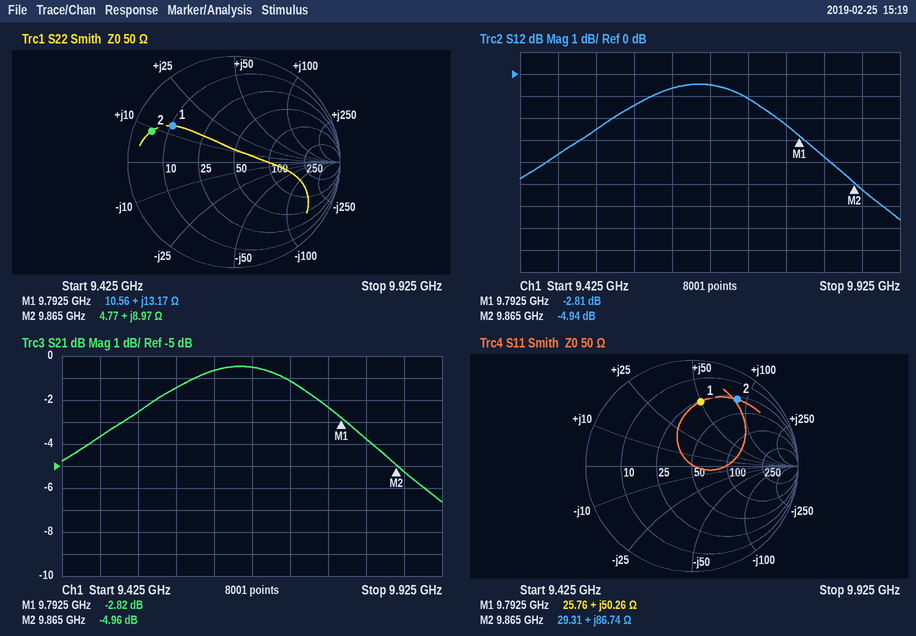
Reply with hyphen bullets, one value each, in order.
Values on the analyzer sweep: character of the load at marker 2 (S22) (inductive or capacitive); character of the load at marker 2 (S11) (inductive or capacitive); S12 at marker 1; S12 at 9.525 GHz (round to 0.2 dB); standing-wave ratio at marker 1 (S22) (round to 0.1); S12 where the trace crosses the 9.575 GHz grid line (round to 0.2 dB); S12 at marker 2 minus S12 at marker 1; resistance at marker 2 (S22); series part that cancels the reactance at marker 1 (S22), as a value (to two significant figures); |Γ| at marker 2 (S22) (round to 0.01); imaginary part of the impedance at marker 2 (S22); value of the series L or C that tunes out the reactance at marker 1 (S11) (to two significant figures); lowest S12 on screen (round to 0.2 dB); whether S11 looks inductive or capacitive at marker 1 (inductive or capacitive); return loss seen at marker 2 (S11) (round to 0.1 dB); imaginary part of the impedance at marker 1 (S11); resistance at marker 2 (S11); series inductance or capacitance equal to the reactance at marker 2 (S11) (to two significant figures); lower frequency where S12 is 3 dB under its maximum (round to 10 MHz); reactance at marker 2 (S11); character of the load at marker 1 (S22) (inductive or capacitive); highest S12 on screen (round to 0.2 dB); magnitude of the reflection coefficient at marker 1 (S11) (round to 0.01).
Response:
- inductive
- inductive
- -2.81 dB
- -2.6 dB
- 5.1
- -1.4 dB
- -2.13 dB
- 4.77 Ω
- 1.2 pF
- 0.83
- +8.97 Ω
- 320 fF
- -6.6 dB
- inductive
- 2.4 dB
- +50.26 Ω
- 29.31 Ω
- 1.4 nH
- 9.48 GHz
- +86.74 Ω
- inductive
- -0.4 dB
- 0.61
